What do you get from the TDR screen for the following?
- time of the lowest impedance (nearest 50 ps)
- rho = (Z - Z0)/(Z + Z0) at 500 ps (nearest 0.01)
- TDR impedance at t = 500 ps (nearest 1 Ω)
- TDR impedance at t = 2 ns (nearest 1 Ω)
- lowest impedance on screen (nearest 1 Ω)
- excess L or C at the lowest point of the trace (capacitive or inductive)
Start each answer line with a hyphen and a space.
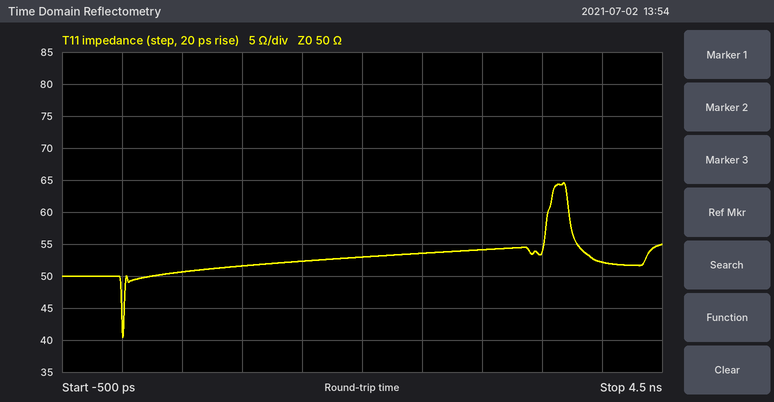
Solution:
- 0 ps
- +0.01
- 51 Ω
- 53 Ω
- 40 Ω
- capacitive
